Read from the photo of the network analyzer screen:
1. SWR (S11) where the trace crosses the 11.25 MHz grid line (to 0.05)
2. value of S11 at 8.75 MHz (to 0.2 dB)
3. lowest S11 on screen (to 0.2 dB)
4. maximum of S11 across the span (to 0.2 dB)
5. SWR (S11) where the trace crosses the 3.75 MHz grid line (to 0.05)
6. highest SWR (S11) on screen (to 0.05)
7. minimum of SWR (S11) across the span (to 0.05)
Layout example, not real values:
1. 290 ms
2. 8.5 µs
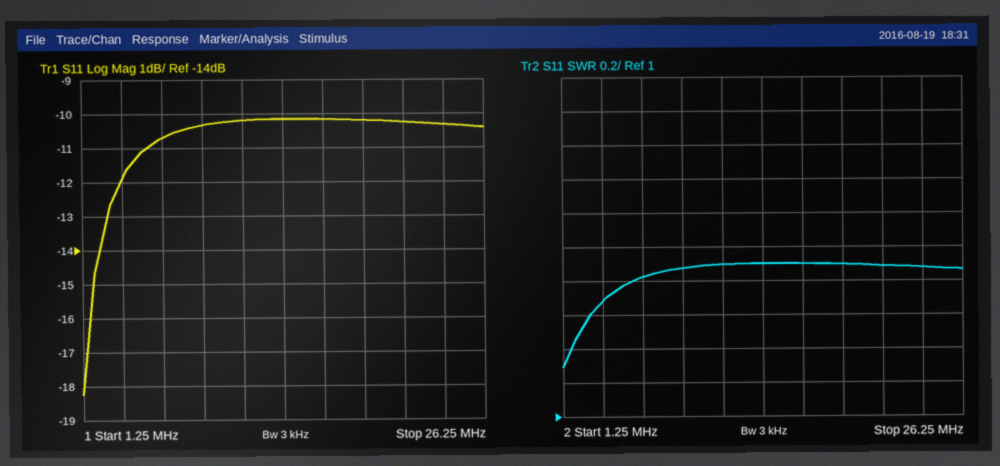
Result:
1. 1.90
2. -10.4 dB
3. -18.2 dB
4. -10.2 dB
5. 1.70
6. 1.90
7. 1.30
